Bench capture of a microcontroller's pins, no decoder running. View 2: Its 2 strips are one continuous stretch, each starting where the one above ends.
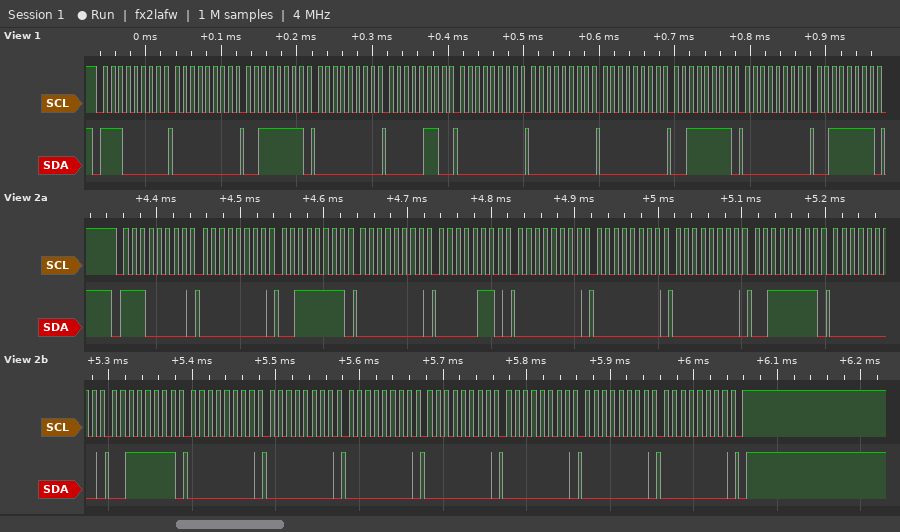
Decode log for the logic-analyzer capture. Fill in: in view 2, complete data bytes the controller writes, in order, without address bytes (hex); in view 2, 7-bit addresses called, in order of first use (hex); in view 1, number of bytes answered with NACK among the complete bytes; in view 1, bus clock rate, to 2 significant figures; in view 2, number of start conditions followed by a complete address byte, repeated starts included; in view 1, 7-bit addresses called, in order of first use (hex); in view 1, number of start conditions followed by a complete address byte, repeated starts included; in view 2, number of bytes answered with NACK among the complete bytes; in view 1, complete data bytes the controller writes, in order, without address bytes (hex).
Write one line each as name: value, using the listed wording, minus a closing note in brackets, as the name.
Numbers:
in view 2, complete data bytes the controller writes, in order, without address bytes: 00 3F 00 06 00 00 00 3F 00 3F 00 00 00 00 00 00 00
in view 2, 7-bit addresses called, in order of first use: 0x70
in view 1, number of bytes answered with NACK among the complete bytes: 0
in view 1, bus clock rate, to 2 significant figures: 100 kHz
in view 2, number of start conditions followed by a complete address byte, repeated starts included: 1
in view 1, 7-bit addresses called, in order of first use: 0x70
in view 1, number of start conditions followed by a complete address byte, repeated starts included: 1
in view 2, number of bytes answered with NACK among the complete bytes: 0
in view 1, complete data bytes the controller writes, in order, without address bytes: 00 3F 00 06 00 00 00 3F 00 3F
